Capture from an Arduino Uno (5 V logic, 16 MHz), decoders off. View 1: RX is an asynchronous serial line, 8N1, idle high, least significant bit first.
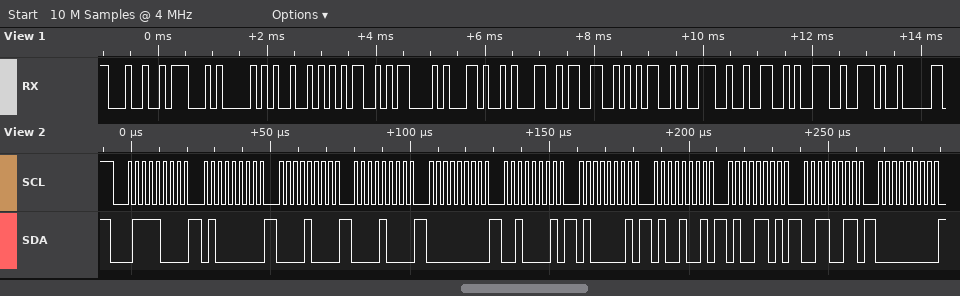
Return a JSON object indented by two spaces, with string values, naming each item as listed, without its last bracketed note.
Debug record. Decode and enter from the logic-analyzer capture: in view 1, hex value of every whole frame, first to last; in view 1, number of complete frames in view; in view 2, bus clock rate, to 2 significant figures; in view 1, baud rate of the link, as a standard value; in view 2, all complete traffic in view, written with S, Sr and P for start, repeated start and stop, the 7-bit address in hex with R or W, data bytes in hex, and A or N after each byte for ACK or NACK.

{
  "in view 1, hex value of every whole frame, first to last": "24 47 50 52 4D 43 2C 31 33 35 39 32 39 2E",
  "in view 1, number of complete frames in view": "14",
  "in view 2, bus clock rate, to 2 significant figures": "400 kHz",
  "in view 1, baud rate of the link, as a standard value": "9600 baud",
  "in view 2, all complete traffic in view, written with S, Sr and P for start, repeated start and stop, the 7-bit address in hex with R or W, data bytes in hex, and A or N after each byte for ACK or NACK": "S 3CW A 40 A 08 A 08 A 00 A 21 A 41 A 49 A 4D A 33 A 00 A"
}
